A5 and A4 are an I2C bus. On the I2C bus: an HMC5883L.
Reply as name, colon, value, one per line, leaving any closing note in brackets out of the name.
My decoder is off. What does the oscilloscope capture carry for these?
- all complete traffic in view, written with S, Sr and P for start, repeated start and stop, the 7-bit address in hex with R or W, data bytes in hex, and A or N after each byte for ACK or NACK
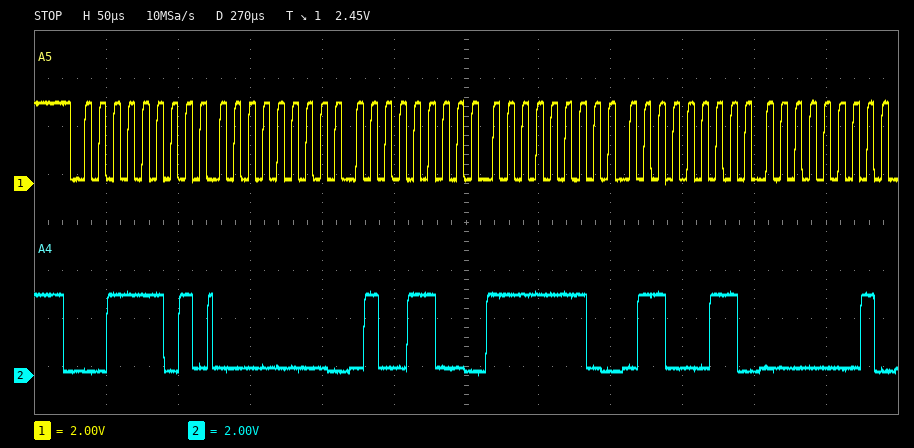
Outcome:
all complete traffic in view, written with S, Sr and P for start, repeated start and stop, the 7-bit address in hex with R or W, data bytes in hex, and A or N after each byte for ACK or NACK: S 1ER A 00 A 4C A FE A 63 A 01 A
